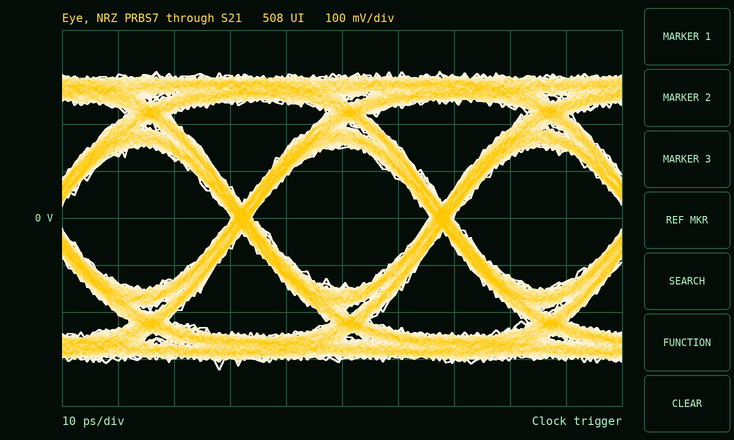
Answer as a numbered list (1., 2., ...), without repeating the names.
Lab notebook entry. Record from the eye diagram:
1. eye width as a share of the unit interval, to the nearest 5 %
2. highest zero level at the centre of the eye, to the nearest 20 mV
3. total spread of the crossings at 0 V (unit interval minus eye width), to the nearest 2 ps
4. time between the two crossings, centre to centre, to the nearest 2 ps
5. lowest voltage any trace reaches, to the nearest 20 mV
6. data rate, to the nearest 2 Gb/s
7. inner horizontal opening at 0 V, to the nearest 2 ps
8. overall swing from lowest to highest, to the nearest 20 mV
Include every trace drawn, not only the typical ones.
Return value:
1. 90 %
2. -140 mV
3. 4 ps
4. 36 ps
5. -320 mV
6. 28 Gb/s
7. 32 ps
8. 640 mV
